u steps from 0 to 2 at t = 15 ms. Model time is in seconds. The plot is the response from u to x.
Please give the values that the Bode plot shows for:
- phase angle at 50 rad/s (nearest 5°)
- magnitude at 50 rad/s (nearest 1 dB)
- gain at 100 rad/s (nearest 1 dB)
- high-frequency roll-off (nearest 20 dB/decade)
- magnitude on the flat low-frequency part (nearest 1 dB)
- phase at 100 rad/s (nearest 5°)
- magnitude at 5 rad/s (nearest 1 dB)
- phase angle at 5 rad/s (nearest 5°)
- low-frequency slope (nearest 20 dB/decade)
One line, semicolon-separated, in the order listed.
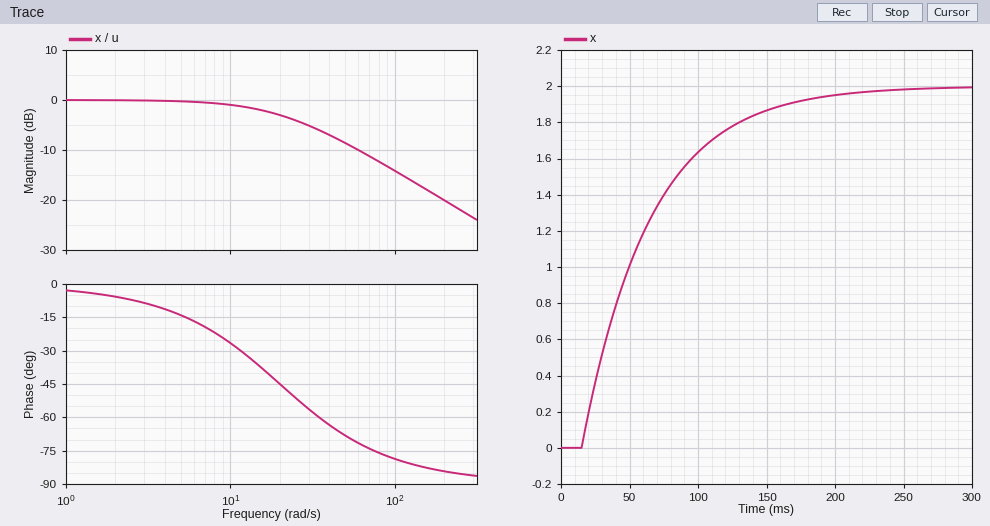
-70°; -9 dB; -14 dB; -20 dB/decade; 0 dB; -80°; 0 dB; -15°; 0 dB/decade
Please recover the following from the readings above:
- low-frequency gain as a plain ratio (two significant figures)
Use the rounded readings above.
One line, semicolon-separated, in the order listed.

1.0
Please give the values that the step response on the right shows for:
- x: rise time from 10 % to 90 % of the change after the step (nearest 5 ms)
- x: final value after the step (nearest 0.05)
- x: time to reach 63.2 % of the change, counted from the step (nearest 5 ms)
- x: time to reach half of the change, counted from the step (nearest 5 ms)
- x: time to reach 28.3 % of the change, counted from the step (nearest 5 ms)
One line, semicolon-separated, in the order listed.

110 ms; 2.00; 50 ms; 35 ms; 15 ms
